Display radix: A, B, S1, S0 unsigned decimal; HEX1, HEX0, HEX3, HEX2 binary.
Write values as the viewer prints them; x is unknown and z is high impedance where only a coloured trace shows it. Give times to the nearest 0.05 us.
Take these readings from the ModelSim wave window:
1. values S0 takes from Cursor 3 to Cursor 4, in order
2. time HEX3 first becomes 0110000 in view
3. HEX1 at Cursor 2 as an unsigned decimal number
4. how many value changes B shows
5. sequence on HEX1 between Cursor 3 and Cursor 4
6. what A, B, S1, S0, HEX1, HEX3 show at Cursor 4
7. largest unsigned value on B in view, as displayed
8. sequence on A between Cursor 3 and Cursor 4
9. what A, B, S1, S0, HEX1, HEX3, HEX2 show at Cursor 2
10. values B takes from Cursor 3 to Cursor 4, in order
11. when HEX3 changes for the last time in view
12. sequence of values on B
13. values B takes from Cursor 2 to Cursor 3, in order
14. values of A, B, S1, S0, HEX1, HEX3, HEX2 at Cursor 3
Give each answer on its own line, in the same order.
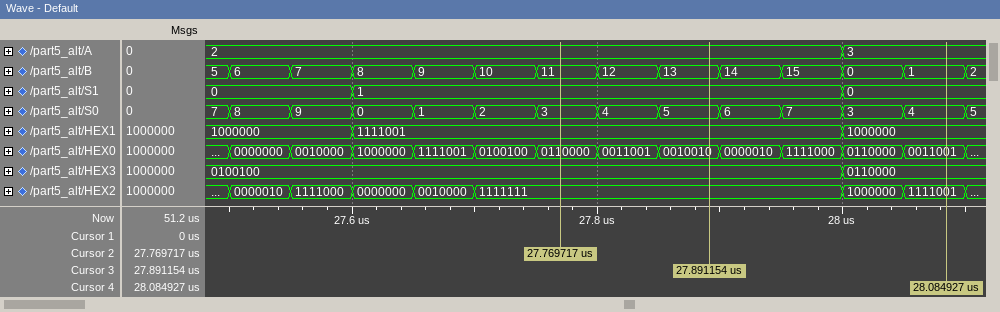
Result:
5, 6, 7, 3, 4
28 us
121
13
1111001, 1000000
A=3, B=1, S1=0, S0=4, HEX1=1000000, HEX3=0110000
15
2, 3
A=2, B=11, S1=1, S0=3, HEX1=1111001, HEX3=0100100, HEX2=1111111
13, 14, 15, 0, 1
28 us
5, 6, 7, 8, 9, 10, 11, 12, 13, 14, 15, 0, 1, 2
11, 12, 13
A=2, B=13, S1=1, S0=5, HEX1=1111001, HEX3=0100100, HEX2=1111111
